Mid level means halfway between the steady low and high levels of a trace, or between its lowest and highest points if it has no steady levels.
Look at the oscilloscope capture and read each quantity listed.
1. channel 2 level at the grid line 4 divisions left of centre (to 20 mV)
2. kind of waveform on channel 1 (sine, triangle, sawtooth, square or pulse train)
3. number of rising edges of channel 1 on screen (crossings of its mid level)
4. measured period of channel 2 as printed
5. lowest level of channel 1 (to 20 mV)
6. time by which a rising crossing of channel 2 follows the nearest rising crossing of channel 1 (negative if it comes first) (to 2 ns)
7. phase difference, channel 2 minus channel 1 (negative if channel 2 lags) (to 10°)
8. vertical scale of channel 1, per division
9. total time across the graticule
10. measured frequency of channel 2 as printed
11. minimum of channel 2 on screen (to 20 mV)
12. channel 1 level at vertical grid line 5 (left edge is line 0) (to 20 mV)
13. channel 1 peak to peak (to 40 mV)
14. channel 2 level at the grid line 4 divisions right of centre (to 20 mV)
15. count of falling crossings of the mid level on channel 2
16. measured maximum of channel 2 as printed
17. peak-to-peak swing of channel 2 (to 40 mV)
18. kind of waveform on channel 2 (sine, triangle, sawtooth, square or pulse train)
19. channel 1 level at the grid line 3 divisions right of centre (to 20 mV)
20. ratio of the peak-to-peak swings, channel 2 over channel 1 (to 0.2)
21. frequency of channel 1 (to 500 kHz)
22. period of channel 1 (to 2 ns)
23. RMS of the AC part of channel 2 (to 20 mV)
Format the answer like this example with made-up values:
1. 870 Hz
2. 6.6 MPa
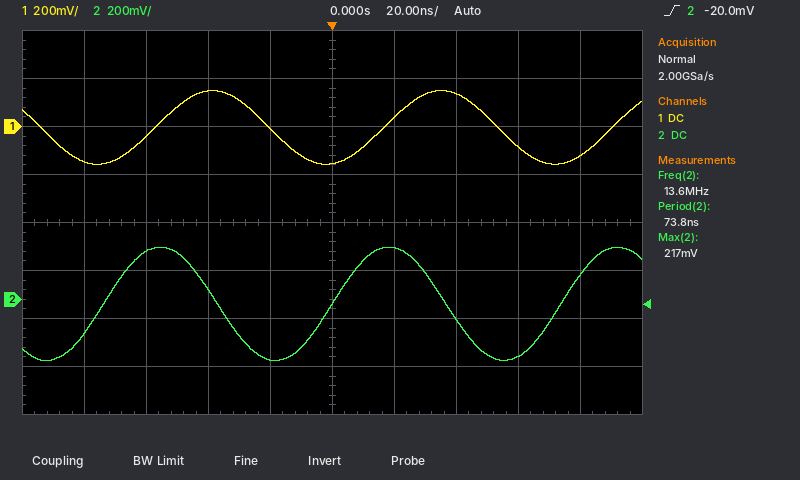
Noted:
1. -140 mV
2. sine
3. 3
4. 73.8 ns
5. -160 mV
6. -16 ns
7. +80°
8. 200 mV
9. 200 ns
10. 13.6 MHz
11. -260 mV
12. -160 mV
13. 320 mV
14. 100 mV
15. 2
16. 217 mV
17. 480 mV
18. sine
19. -80 mV
20. 1.6
21. 13.5 MHz
22. 74 ns
23. 160 mV
